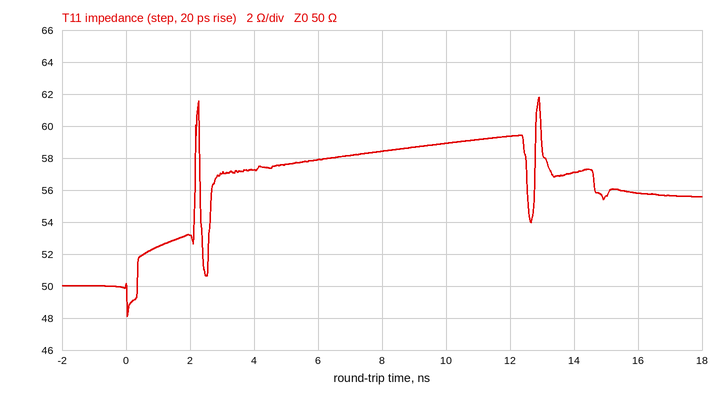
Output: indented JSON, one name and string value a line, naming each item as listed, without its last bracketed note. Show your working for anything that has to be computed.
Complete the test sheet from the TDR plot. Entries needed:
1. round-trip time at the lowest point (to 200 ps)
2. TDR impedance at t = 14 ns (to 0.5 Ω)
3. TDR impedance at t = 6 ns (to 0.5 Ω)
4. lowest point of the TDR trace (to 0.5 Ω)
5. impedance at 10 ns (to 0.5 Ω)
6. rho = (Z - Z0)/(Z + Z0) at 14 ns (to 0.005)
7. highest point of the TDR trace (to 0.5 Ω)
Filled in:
{
  "round-trip time at the lowest point": "0.0 ns",
  "TDR impedance at t = 14 ns": "57.0 Ω",
  "TDR impedance at t = 6 ns": "58.0 Ω",
  "lowest point of the TDR trace": "48.0 Ω",
  "impedance at 10 ns": "59.0 Ω",
  "rho = (Z - Z0)/(Z + Z0) at 14 ns": "(57 − 50)/(57 + 50) ≈ +0.065",
  "highest point of the TDR trace": "62.0 Ω"
}
